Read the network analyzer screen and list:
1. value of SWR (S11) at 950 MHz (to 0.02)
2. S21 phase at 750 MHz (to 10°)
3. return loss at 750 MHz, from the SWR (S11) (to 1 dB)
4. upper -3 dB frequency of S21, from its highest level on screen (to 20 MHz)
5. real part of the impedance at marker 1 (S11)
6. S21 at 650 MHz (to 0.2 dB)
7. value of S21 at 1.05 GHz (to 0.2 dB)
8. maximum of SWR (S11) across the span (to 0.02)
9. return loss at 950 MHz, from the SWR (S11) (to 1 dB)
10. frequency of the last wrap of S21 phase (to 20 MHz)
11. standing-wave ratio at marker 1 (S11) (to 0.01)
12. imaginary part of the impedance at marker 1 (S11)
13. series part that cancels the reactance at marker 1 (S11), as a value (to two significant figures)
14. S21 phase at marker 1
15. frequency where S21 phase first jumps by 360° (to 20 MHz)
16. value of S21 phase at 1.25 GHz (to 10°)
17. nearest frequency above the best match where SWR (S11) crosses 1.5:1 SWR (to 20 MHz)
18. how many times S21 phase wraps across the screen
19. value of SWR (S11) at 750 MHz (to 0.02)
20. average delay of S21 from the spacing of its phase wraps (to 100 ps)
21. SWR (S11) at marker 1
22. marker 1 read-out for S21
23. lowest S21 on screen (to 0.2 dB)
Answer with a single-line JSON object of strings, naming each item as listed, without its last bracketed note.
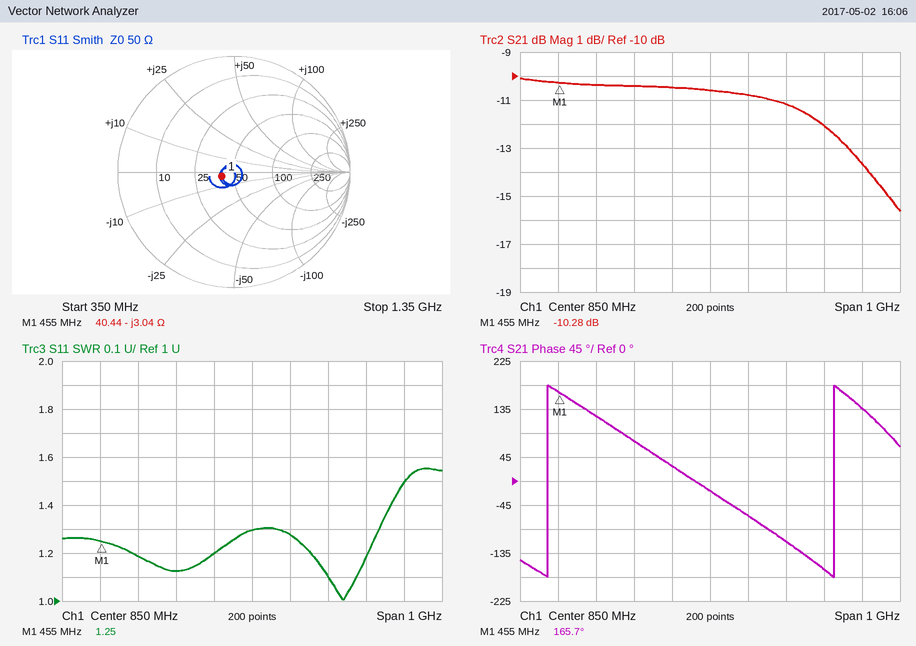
{"value of SWR (S11) at 950 MHz": "1.28", "S21 phase at 750 MHz": "30°", "return loss at 750 MHz, from the SWR (S11)": "21 dB", "upper -3 dB frequency of S21, from its highest level on screen": "1.22 GHz", "real part of the impedance at marker 1": "40.44 Ω", "S21 at 650 MHz": "-10.4 dB", "value of S21 at 1.05 GHz": "-11.2 dB", "maximum of SWR (S11) across the span": "1.56", "return loss at 950 MHz, from the SWR (S11)": "18 dB", "frequency of the last wrap of S21 phase": "1.18 GHz", "standing-wave ratio at marker 1 (S11)": "1.25", "imaginary part of the impedance at marker 1": "-3.04 Ω", "series part that cancels the reactance at marker 1 (S11), as a value": "1.1 nH", "S21 phase at marker 1": "165.7°", "frequency where S21 phase first jumps by 360°": "420 MHz", "value of S21 phase at 1.25 GHz": "140°", "nearest frequency above the best match where SWR (S11) crosses 1.5:1 SWR": "1.26 GHz", "how many times S21 phase wraps across the screen": "2", "value of SWR (S11) at 750 MHz": "1.20", "average delay of S21 from the spacing of its phase wraps": "1.3 ns", "SWR (S11) at marker 1": "1.25", "marker 1 read-out for S21": "-10.28 dB", "lowest S21 on screen": "-15.6 dB"}
